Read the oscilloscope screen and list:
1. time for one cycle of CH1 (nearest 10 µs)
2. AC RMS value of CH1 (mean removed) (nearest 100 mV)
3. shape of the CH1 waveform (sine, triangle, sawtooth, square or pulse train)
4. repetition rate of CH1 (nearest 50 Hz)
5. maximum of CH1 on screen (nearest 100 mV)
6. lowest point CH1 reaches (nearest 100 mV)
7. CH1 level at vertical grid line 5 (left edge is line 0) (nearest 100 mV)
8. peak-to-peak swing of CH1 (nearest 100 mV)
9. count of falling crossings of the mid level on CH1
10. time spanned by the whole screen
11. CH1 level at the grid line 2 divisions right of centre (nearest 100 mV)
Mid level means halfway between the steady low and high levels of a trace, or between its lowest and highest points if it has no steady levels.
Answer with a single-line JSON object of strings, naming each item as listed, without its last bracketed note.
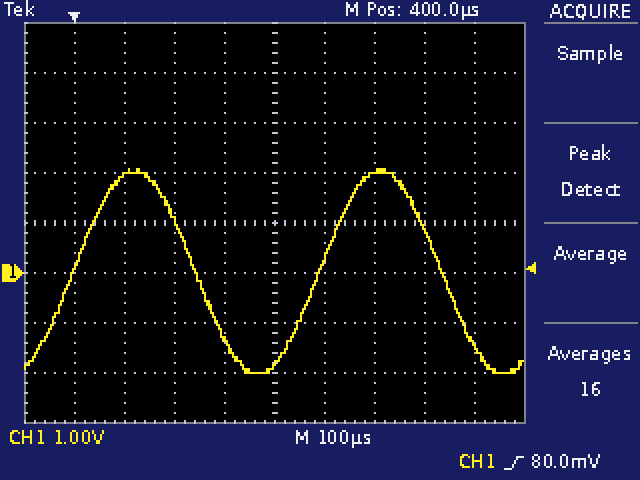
{"time for one cycle of CH1": "490 µs", "AC RMS value of CH1 (mean removed)": "1.4 V", "shape of the CH1 waveform": "sine", "repetition rate of CH1": "2.05 kHz", "maximum of CH1 on screen": "2.1 V", "lowest point CH1 reaches": "-2.0 V", "CH1 level at vertical grid line 5 (left edge is line 0)": "-1.8 V", "peak-to-peak swing of CH1": "4.1 V", "count of falling crossings of the mid level on CH1": "2", "time spanned by the whole screen": "1 ms", "CH1 level at the grid line 2 divisions right of centre": "2.0 V"}
